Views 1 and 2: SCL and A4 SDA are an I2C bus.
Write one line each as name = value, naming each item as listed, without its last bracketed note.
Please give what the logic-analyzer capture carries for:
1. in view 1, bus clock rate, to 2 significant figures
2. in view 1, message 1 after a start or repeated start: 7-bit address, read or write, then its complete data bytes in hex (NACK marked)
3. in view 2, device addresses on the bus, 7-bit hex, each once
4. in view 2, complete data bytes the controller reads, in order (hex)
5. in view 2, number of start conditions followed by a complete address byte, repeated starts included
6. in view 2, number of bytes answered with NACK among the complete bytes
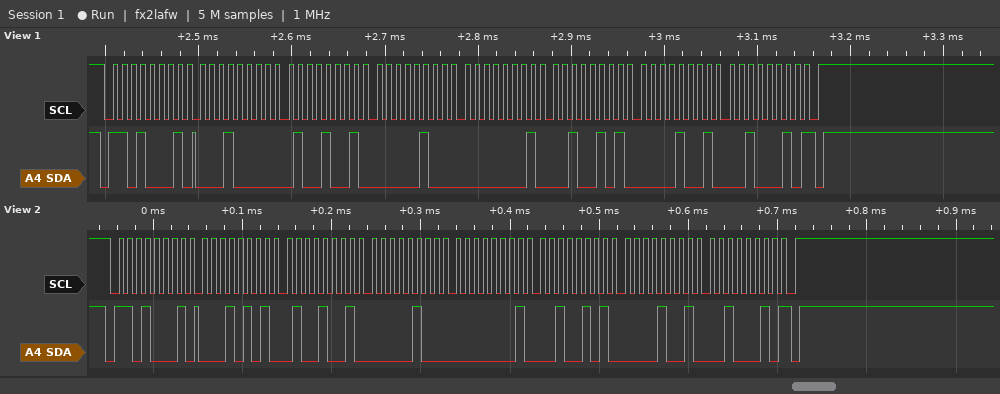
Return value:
in view 1, bus clock rate, to 2 significant figures = 100 kHz
in view 1, message 1 after a start or repeated start: 7-bit address, read or write, then its complete data bytes in hex = 0x68 read: 10 49 04 01 25 09 22 NACK
in view 2, device addresses on the bus, 7-bit hex, each once = 0x68
in view 2, complete data bytes the controller reads, in order = 15 49 04 01 25 09 22
in view 2, number of start conditions followed by a complete address byte, repeated starts included = 1
in view 2, number of bytes answered with NACK among the complete bytes = 1
